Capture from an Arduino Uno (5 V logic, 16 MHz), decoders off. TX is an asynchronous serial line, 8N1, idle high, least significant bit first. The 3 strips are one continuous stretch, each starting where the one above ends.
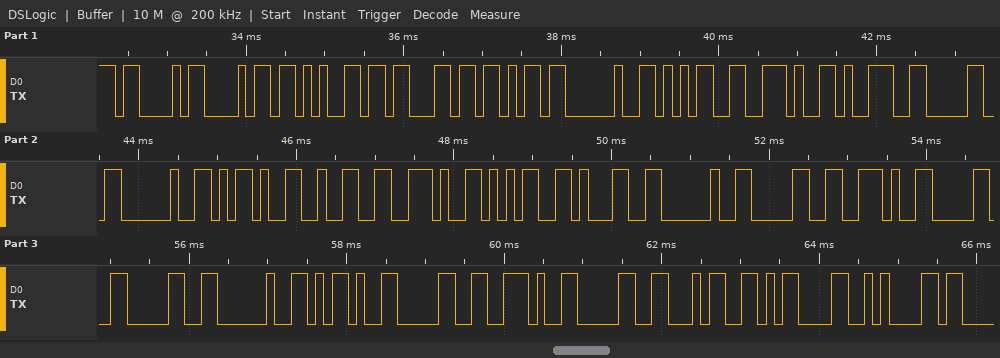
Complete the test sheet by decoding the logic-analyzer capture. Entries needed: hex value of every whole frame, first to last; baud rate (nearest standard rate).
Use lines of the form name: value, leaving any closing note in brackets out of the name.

hex value of every whole frame, first to last: 0x43 0x68 0x65 0x63 0x6B 0x20 0x35 0x2E 0x39 0x30 0x20 0x2D 0x32 0x2E 0x35 0x31 0x20 0x30 0x2E 0x30 0x30 0x20 0x2D 0x30 0x2E 0x30 0x34 0x0D 0x0A
baud rate: 9600 baud
